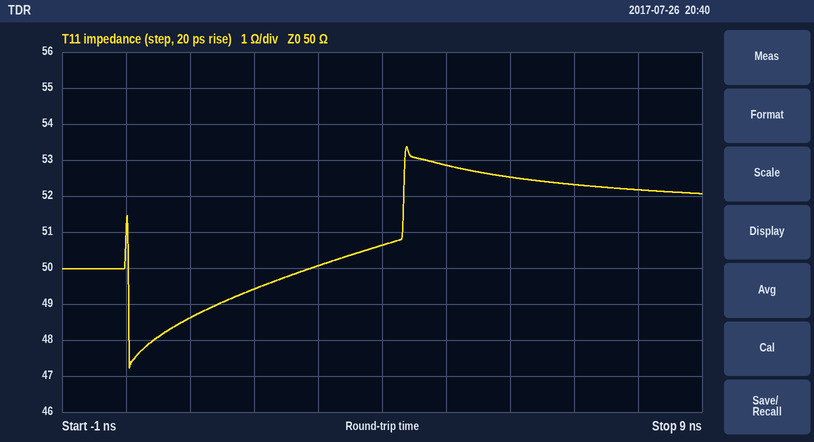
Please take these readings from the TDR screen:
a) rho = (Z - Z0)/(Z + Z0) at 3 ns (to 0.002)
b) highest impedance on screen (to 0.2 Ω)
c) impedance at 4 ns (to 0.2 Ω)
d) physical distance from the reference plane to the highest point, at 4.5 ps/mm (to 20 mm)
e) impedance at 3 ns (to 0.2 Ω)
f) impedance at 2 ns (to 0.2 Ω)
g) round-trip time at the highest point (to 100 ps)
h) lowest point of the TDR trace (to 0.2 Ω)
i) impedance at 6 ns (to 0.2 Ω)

0.000
53.4 Ω
50.6 Ω
480 mm
50.0 Ω
49.4 Ω
4.4 ns
47.2 Ω
52.6 Ω
